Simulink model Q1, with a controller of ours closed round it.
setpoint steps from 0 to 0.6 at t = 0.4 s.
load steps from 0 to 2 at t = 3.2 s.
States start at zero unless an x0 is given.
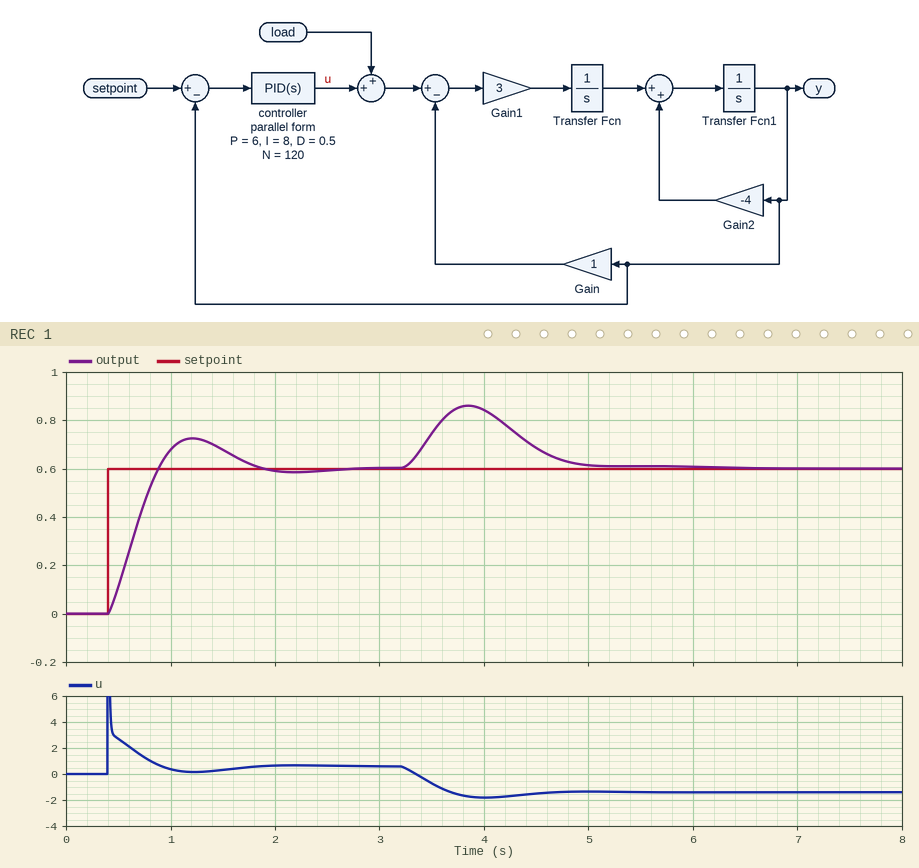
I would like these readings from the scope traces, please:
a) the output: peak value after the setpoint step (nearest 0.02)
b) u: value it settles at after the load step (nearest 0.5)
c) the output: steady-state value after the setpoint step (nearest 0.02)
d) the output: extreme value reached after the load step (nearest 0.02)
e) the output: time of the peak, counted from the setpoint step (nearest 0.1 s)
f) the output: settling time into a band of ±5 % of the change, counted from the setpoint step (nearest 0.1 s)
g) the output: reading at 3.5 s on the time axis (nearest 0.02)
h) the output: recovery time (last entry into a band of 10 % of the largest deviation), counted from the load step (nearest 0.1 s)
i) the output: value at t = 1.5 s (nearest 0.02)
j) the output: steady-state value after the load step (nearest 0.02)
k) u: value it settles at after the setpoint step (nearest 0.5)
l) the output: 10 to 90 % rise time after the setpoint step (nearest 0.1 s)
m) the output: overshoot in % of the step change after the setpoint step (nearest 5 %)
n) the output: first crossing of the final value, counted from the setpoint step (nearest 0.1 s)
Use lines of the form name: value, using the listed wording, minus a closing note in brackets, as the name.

the output: peak value after the setpoint step: 0.72
u: value it settles at after the load step: -1.5
the output: steady-state value after the setpoint step: 0.60
the output: extreme value reached after the load step: 0.86
the output: time of the peak, counted from the setpoint step: 0.8 s
the output: settling time into a band of ±5 % of the change, counted from the setpoint step: 1.3 s
the output: reading at 3.5 s on the time axis: 0.74
the output: recovery time (last entry into a band of 10 % of the largest deviation), counted from the load step: 1.6 s
the output: value at t = 1.5 s: 0.68
the output: steady-state value after the load step: 0.60
u: value it settles at after the setpoint step: 0.5
the output: 10 to 90 % rise time after the setpoint step: 0.4 s
the output: overshoot in % of the step change after the setpoint step: 20 %
the output: first crossing of the final value, counted from the setpoint step: 0.5 s
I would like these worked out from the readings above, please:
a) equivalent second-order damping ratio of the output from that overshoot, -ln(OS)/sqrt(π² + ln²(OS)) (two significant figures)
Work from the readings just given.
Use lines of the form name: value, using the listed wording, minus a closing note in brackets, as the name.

equivalent second-order damping ratio of the output from that overshoot, -ln(OS)/sqrt(π² + ln²(OS)): 0.46
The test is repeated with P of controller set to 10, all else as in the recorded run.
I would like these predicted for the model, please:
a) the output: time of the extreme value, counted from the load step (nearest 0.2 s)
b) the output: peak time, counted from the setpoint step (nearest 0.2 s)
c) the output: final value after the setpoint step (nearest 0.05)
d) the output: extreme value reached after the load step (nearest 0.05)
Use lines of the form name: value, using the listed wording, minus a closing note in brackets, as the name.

the output: time of the extreme value, counted from the load step: 0.6 s
the output: peak time, counted from the setpoint step: 0.6 s
the output: final value after the setpoint step: 0.60
the output: extreme value reached after the load step: 0.80
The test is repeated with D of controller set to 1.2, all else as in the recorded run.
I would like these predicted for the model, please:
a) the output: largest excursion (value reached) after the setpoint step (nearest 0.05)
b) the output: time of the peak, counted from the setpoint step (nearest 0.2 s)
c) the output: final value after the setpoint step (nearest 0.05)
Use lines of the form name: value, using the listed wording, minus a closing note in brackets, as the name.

the output: largest excursion (value reached) after the setpoint step: 0.65
the output: time of the peak, counted from the setpoint step: 1.0 s
the output: final value after the setpoint step: 0.60
